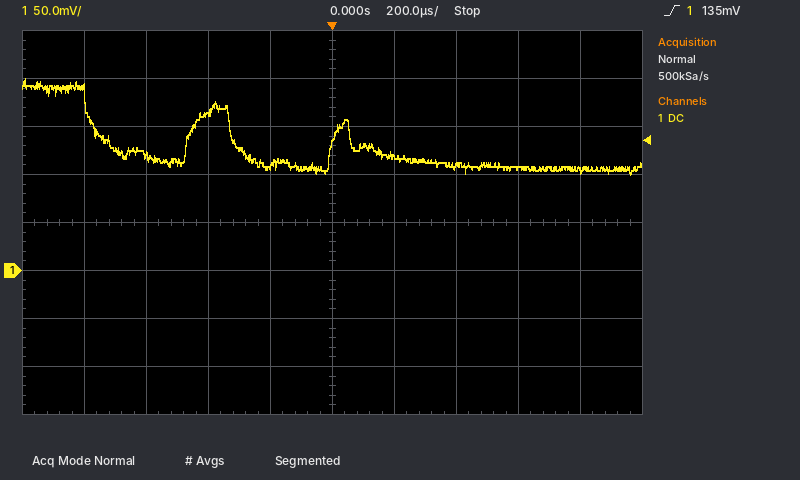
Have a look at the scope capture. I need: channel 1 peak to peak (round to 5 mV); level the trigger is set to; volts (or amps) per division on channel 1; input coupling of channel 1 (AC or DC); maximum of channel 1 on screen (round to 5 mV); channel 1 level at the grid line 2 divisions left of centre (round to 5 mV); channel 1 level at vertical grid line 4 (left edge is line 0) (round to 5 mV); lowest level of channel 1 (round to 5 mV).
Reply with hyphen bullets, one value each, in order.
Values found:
- 100 mV
- 135 mV
- 50 mV
- DC
- 200 mV
- 165 mV
- 110 mV
- 100 mV
